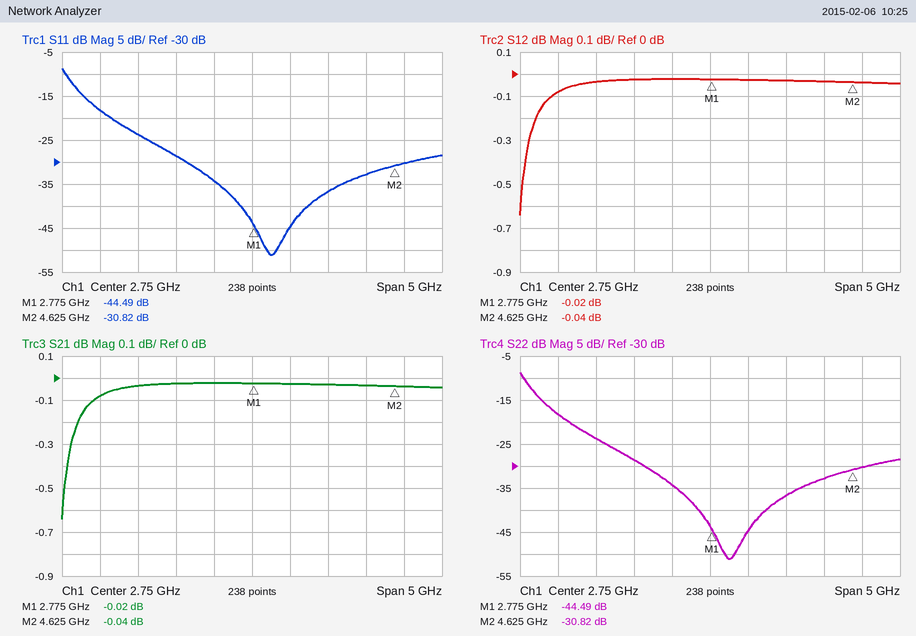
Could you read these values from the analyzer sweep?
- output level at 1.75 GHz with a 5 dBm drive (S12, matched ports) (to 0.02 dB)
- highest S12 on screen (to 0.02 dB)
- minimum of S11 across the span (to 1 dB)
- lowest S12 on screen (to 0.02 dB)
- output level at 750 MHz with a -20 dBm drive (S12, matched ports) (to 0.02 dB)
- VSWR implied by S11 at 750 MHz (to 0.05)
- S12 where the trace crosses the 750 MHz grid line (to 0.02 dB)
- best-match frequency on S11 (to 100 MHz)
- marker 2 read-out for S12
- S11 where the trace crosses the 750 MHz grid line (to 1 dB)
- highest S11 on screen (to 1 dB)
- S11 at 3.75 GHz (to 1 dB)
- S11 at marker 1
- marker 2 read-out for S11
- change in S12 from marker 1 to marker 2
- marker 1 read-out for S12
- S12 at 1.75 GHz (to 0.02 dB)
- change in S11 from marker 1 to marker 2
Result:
4.98 dBm
-0.02 dB
-51 dB
-0.64 dB
-20.08 dBm
1.30
-0.08 dB
3.0 GHz
-0.04 dB
-18 dB
-9 dB
-37 dB
-44.49 dB
-30.82 dB
-0.02 dB
-0.02 dB
-0.02 dB
13.67 dB
